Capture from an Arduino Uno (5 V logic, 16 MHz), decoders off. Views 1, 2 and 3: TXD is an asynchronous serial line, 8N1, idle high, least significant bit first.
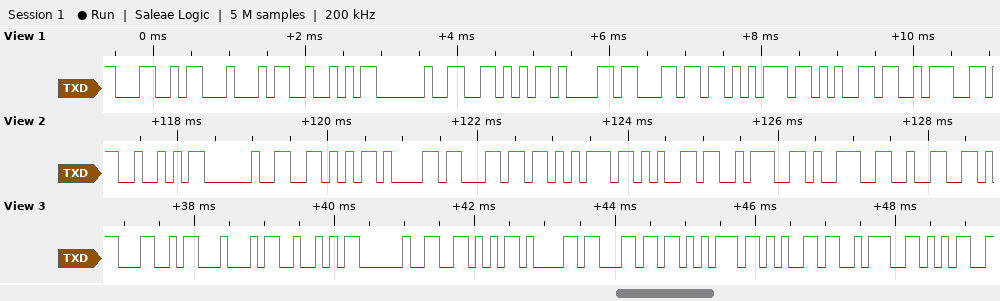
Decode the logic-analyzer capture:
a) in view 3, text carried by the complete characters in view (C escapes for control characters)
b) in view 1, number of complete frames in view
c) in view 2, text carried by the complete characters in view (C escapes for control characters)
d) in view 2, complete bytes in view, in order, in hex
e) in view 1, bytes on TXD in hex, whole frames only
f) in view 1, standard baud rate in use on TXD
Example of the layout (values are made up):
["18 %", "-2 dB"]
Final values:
["\"LDR Value:5\"", "10", "\"R Value:92\"", "0x52 0x20 0x56 0x61 0x6C 0x75 0x65 0x3A 0x39 0x32", "4C 44 52 20 56 61 6C 75 65 3A", "9600 baud"]
